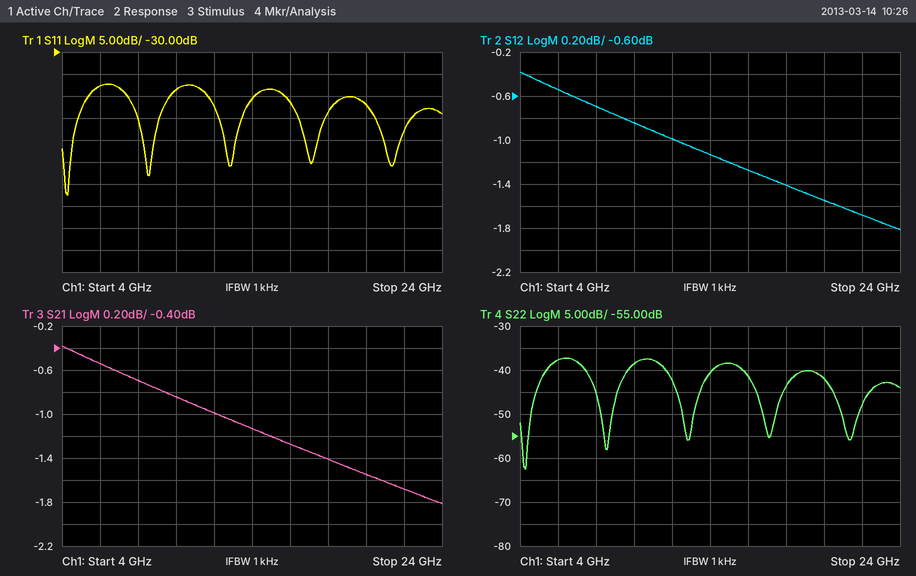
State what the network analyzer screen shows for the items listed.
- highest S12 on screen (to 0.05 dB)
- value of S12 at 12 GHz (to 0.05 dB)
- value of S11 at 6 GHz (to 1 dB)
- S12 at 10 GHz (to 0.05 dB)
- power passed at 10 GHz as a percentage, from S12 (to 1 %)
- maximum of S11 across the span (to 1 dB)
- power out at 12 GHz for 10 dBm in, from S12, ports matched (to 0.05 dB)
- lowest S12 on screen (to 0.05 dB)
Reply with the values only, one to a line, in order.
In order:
-0.40 dB
-1.00 dB
-38 dB
-0.85 dB
82 %
-37 dB
9.00 dBm
-1.80 dB
